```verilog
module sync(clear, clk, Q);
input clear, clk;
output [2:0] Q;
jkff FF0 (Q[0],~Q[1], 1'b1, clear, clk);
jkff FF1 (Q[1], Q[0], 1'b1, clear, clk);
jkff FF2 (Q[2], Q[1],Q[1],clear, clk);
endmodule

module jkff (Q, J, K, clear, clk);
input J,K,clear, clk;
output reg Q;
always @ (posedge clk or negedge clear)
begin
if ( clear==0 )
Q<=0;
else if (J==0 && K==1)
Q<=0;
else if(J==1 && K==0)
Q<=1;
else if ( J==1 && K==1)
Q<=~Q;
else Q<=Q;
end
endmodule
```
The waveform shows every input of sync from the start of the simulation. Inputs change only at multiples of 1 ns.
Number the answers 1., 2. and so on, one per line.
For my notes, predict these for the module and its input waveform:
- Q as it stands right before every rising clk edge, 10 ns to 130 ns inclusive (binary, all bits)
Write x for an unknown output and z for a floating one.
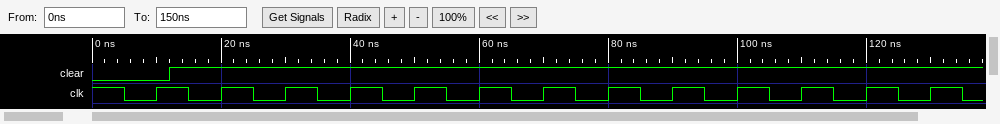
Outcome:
1. 000, 000, 001, 010, 100, 101, 110, 000, 001, 010, 100, 101, 110
